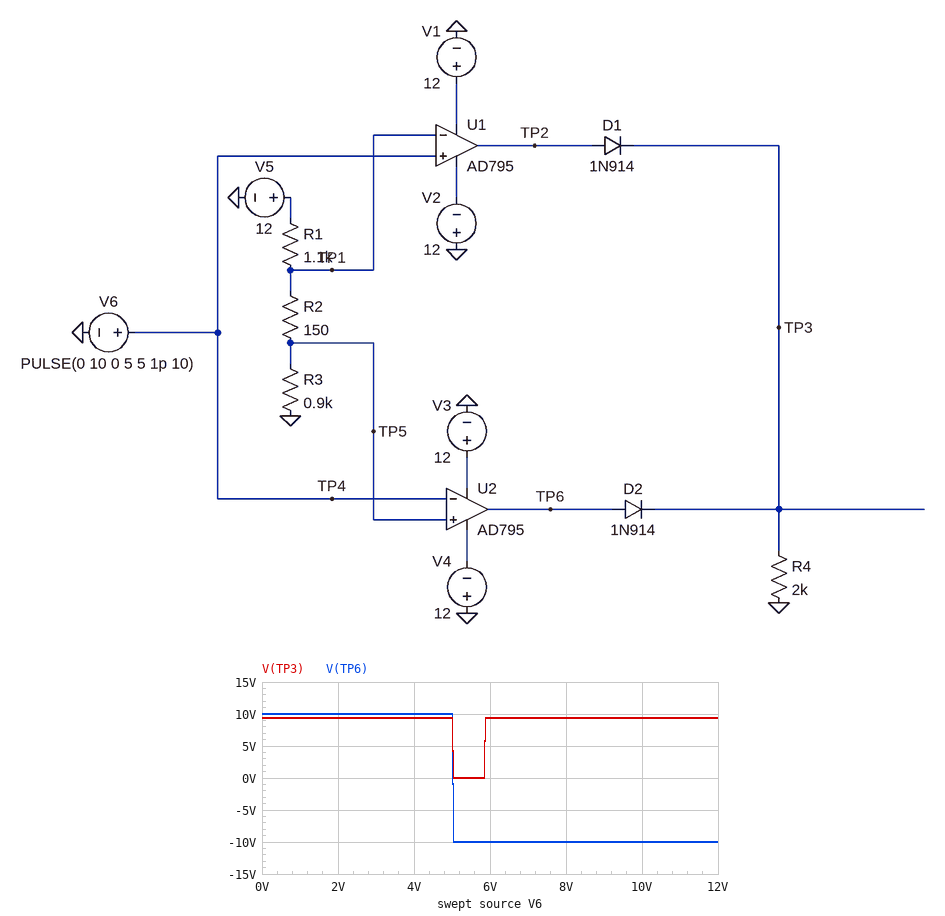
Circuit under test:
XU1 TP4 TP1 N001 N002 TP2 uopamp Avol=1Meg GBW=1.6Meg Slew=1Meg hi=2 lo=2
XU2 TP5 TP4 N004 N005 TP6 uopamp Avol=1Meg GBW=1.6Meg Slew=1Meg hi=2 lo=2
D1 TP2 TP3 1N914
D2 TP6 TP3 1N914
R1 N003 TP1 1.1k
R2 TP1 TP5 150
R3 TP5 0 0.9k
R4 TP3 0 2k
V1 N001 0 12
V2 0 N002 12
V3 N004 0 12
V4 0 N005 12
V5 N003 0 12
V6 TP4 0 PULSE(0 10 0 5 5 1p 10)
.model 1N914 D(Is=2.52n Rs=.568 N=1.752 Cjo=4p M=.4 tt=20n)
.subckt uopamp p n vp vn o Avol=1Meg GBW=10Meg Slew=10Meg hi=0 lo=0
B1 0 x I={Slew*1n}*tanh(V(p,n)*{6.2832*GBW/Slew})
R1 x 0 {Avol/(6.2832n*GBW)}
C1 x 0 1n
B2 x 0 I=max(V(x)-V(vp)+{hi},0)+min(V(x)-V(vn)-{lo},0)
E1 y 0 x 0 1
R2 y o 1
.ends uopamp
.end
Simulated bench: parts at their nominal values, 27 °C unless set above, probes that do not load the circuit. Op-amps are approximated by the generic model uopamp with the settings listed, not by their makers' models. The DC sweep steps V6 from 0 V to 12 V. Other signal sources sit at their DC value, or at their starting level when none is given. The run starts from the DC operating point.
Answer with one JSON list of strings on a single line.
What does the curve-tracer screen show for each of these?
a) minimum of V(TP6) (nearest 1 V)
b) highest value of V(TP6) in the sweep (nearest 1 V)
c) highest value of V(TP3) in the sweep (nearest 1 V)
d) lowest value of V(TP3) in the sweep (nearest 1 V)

["-10 V", "10 V", "9 V", "0 V"]
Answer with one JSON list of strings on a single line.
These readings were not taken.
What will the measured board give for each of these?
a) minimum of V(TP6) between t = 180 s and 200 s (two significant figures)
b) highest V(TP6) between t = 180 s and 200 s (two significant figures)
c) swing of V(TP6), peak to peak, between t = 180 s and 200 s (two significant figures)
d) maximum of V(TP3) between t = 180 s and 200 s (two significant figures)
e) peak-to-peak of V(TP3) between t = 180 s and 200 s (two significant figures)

["-10 V", "10 V", "20 V", "9.3 V", "9.3 V"]
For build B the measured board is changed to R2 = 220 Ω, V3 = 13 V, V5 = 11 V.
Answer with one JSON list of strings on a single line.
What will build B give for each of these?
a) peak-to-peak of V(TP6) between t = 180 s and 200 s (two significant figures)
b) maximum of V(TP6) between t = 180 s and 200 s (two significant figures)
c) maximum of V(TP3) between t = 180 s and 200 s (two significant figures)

["21 V", "11 V", "10 V"]
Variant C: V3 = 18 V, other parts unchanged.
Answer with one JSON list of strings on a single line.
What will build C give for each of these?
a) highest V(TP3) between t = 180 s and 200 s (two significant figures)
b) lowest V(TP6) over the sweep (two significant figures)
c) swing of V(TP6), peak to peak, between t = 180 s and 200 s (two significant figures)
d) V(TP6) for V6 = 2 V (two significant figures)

["15 V", "-10 V", "26 V", "16 V"]
